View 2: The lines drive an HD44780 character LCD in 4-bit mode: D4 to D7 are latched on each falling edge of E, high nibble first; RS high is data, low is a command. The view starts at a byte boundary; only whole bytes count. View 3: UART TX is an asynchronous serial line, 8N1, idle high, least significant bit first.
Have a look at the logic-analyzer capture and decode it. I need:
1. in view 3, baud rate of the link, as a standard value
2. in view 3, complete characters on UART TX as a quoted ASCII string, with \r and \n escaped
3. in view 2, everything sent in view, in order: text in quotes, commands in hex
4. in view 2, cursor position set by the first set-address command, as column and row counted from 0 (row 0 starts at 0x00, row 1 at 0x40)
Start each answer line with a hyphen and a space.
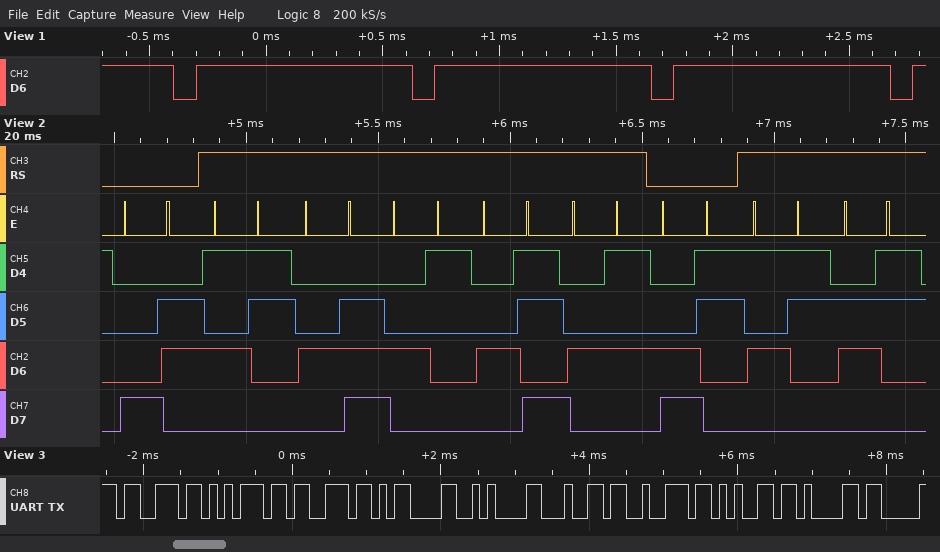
- 9600 baud
- "sus\r\ndrea"
- 0x86 "SNAKE" 0xC3 "Sc"
- column 6, row 0
